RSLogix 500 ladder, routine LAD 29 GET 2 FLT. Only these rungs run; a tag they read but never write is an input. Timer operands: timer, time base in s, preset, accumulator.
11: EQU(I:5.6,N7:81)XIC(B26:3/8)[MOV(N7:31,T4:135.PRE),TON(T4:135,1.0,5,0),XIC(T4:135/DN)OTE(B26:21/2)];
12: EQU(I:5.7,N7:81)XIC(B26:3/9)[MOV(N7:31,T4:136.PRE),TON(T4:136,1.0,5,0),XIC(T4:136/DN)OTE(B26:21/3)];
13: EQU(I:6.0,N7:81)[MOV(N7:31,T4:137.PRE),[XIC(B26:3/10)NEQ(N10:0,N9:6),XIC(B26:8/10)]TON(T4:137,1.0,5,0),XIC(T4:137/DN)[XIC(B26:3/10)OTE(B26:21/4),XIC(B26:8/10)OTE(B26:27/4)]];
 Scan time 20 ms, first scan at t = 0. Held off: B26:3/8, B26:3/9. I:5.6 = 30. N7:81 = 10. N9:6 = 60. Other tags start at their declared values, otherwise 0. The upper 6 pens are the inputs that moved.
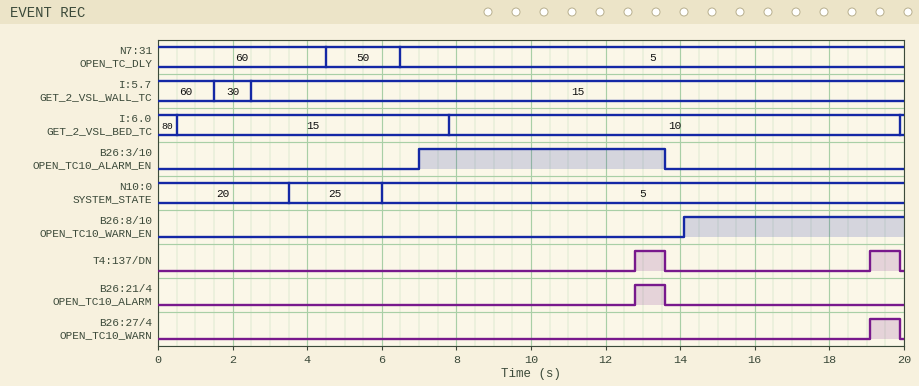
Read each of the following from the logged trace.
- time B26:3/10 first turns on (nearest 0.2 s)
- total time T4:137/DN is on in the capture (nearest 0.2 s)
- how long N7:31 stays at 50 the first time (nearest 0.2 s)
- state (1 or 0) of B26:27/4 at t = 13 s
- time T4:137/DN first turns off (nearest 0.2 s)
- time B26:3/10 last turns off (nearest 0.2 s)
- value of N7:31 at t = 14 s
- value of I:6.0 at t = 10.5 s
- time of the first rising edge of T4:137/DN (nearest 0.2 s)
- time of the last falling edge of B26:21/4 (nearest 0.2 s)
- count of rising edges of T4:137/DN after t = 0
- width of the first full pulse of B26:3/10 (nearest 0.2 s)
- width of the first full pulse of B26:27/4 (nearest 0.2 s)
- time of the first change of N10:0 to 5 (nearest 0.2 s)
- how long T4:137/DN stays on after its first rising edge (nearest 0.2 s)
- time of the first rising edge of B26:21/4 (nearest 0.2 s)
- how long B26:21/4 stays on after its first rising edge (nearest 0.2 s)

7.0 s
1.6 s
2.0 s
0
13.6 s
13.6 s
5
10
12.8 s
13.6 s
2
6.6 s
0.8 s
6.0 s
0.8 s
12.8 s
0.8 s
